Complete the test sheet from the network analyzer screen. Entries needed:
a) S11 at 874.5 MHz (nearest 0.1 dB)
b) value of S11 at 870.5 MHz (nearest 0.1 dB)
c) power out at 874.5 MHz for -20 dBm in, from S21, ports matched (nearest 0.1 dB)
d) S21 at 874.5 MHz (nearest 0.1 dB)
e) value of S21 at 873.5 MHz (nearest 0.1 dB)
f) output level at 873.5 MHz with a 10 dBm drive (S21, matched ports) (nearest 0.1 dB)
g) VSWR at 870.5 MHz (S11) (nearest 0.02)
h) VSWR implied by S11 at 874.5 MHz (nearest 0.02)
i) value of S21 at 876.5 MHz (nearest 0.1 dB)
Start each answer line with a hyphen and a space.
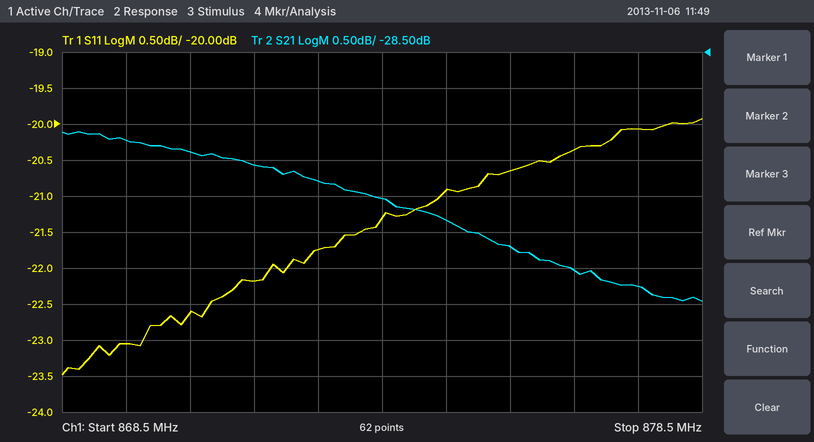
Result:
- -20.9 dB
- -22.6 dB
- -50.8 dBm
- -30.8 dB
- -30.5 dB
- -20.5 dBm
- 1.16
- 1.20
- -31.5 dB
